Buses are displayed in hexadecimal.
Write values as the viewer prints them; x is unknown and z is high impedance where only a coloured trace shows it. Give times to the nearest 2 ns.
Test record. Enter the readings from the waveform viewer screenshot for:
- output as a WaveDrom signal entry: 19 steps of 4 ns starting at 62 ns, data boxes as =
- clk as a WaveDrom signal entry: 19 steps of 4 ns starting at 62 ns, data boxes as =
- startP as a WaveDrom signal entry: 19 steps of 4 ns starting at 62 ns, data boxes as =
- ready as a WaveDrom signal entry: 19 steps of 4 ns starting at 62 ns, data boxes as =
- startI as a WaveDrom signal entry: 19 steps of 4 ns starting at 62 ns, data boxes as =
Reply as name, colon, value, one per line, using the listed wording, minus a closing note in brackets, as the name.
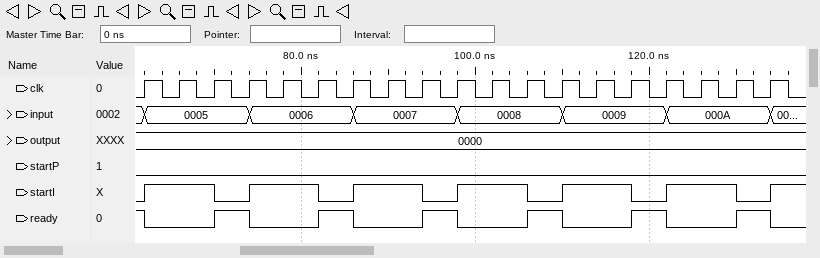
output as a WaveDrom signal entry: 19 steps of 4 ns starting at 62 ns, data boxes as =: {name: 'output', wave: '=..................', data: '0000'}
clk as a WaveDrom signal entry: 19 steps of 4 ns starting at 62 ns, data boxes as =: {name: 'clk', wave: 'p..................'}
startP as a WaveDrom signal entry: 19 steps of 4 ns starting at 62 ns, data boxes as =: {name: 'startP', wave: '0..................'}
ready as a WaveDrom signal entry: 19 steps of 4 ns starting at 62 ns, data boxes as =: {name: 'ready', wave: '0.10.10.10.10.10.10'}
startI as a WaveDrom signal entry: 19 steps of 4 ns starting at 62 ns, data boxes as =: {name: 'startI', wave: '1.01.01.01.01.01.01'}
